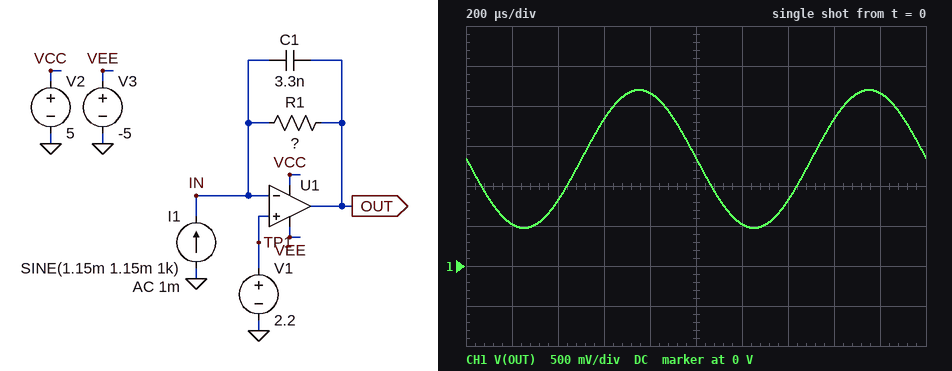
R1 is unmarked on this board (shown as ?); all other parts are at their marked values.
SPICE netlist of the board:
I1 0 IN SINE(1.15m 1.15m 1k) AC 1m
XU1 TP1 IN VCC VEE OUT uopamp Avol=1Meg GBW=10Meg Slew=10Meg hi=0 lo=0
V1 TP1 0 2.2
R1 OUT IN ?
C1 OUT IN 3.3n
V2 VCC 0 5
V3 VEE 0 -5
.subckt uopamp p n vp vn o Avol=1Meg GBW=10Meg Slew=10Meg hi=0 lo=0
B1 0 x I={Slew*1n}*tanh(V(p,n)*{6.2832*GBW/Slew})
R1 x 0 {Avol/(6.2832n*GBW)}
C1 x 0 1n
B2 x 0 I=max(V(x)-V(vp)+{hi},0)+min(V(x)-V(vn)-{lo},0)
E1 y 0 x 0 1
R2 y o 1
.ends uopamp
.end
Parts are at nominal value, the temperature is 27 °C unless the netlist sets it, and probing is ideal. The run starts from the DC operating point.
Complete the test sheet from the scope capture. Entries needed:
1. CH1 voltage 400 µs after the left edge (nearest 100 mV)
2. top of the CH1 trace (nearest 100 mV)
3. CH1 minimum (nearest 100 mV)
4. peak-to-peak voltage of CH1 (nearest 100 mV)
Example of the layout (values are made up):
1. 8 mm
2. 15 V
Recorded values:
1. 800 mV
2. 2.2 V
3. 500 mV
4. 1.7 V
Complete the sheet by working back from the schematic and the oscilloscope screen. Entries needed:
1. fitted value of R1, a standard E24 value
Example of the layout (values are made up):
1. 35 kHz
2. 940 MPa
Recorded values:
1. 750 Ω
